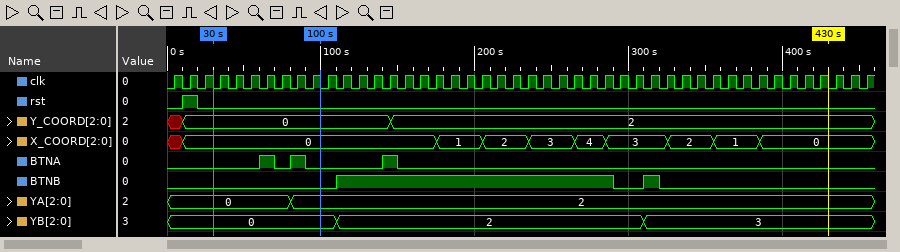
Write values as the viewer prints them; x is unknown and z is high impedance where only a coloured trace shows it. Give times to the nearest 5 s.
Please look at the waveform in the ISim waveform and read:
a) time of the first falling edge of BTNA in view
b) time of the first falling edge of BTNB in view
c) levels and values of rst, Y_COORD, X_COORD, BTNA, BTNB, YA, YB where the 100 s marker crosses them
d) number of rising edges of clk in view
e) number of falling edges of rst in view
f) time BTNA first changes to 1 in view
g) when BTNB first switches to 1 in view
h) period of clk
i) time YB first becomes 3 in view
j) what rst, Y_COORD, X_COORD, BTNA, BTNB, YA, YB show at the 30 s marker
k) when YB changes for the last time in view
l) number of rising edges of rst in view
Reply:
70 s
290 s
rst=0, Y_COORD=0, X_COORD=0, BTNA=0, BTNB=0, YA=2, YB=0
46
1
60 s
110 s
10 s
310 s
rst=0, Y_COORD=0, X_COORD=0, BTNA=0, BTNB=0, YA=0, YB=0
310 s
1
